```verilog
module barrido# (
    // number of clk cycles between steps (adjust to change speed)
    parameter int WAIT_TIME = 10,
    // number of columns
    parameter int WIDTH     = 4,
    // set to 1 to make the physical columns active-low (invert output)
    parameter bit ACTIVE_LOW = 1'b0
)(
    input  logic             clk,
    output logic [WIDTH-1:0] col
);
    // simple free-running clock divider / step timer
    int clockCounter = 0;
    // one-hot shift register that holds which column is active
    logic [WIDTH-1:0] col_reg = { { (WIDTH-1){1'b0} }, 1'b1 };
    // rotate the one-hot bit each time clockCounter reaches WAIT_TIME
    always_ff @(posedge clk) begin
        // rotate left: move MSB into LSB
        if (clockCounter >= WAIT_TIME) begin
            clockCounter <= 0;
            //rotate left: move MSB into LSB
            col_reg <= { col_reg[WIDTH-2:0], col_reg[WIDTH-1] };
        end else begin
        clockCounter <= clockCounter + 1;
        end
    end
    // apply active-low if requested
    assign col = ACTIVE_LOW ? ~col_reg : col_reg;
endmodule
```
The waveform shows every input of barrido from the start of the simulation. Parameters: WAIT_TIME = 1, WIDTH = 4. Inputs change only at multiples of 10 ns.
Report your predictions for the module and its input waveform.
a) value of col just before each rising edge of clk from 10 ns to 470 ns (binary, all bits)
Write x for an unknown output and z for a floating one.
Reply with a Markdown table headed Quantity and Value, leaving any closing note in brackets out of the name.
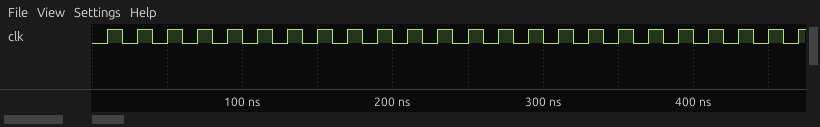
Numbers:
| Quantity | Value |
|---|---|
| value of col just before each rising edge of clk from 10 ns to 470 ns | 0001, 0001, 0010, 0010, 0100, 0100, 1000, 1000, 0001, 0001, 0010, 0010, 0100, 0100, 1000, 1000, 0001, 0001, 0010, 0010, 0100, 0100, 1000, 1000 |
